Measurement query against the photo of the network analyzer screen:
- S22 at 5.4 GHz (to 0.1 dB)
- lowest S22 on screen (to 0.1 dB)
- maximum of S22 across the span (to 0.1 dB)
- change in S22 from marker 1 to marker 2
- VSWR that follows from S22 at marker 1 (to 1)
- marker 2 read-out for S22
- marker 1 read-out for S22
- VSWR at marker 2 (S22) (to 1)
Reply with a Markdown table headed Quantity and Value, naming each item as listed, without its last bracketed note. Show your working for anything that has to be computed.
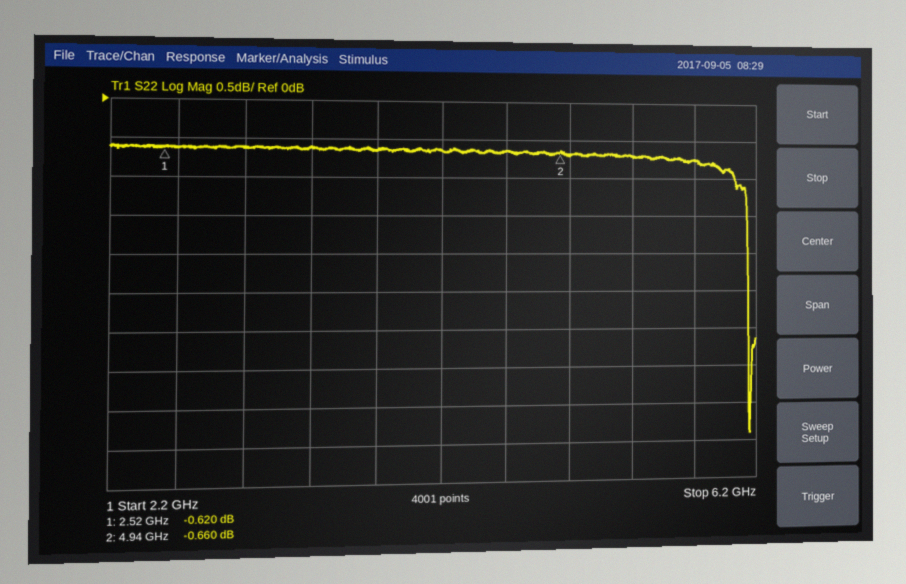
| Quantity | Value |
|---|---|
| S22 at 5.4 GHz | -0.7 dB |
| lowest S22 on screen | -4.4 dB |
| maximum of S22 across the span | -0.6 dB |
| change in S22 from marker 1 to marker 2 | -0.66 − (-0.62) = -0.040 dB |
| VSWR that follows from S22 at marker 1 | (1 + 0.9311)/(1 − 0.9311) ≈ 28 |
| marker 2 read-out for S22 | -0.660 dB |
| marker 1 read-out for S22 | -0.620 dB |
| VSWR at marker 2 (S22) | (1 + 0.9268)/(1 − 0.9268) ≈ 26 |
